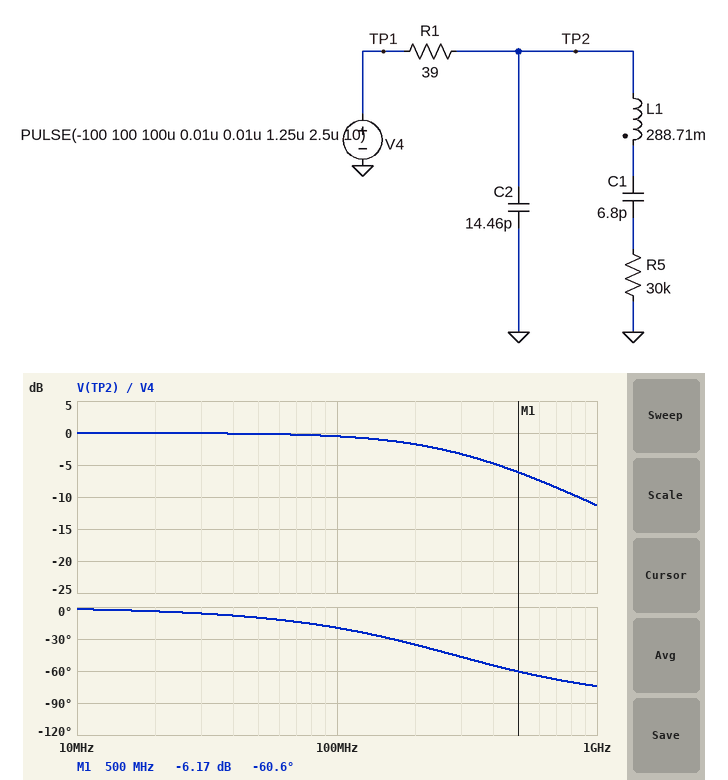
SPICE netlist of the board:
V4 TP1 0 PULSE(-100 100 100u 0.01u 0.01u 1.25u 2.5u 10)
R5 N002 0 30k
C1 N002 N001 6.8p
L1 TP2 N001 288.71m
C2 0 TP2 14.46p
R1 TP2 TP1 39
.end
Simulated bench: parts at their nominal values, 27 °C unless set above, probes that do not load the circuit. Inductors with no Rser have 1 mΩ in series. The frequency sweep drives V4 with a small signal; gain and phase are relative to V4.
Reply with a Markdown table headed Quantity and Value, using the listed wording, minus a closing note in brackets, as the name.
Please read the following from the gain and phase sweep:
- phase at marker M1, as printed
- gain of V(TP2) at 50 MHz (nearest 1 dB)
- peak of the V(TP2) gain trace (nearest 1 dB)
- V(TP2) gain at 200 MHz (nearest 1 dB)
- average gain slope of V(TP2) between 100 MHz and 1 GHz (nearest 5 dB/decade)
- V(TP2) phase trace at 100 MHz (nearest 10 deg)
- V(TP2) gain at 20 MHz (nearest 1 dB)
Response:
| Quantity | Value |
|---|---|
| phase at marker M1, as printed | -60.6 deg |
| gain of V(TP2) at 50 MHz | 0 dB |
| peak of the V(TP2) gain trace | 0 dB |
| V(TP2) gain at 200 MHz | -2 dB |
| average gain slope of V(TP2) between 100 MHz and 1 GHz | -10 dB/decade |
| V(TP2) phase trace at 100 MHz | -20 deg |
| V(TP2) gain at 20 MHz | 0 dB |
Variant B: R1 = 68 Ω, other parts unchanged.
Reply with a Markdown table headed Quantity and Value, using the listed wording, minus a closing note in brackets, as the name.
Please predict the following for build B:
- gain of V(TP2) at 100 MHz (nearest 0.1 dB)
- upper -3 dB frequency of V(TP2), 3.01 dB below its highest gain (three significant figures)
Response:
| Quantity | Value |
|---|---|
| gain of V(TP2) at 100 MHz | -1.4 dB |
| upper -3 dB frequency of V(TP2), 3.01 dB below its highest gain | 162 MHz |
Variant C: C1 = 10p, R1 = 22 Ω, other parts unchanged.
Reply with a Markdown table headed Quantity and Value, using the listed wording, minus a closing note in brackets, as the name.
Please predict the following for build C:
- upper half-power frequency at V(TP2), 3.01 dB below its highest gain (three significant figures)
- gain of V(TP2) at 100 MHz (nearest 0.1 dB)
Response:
| Quantity | Value |
|---|---|
| upper half-power frequency at V(TP2), 3.01 dB below its highest gain | 500 MHz |
| gain of V(TP2) at 100 MHz | -0.2 dB |
